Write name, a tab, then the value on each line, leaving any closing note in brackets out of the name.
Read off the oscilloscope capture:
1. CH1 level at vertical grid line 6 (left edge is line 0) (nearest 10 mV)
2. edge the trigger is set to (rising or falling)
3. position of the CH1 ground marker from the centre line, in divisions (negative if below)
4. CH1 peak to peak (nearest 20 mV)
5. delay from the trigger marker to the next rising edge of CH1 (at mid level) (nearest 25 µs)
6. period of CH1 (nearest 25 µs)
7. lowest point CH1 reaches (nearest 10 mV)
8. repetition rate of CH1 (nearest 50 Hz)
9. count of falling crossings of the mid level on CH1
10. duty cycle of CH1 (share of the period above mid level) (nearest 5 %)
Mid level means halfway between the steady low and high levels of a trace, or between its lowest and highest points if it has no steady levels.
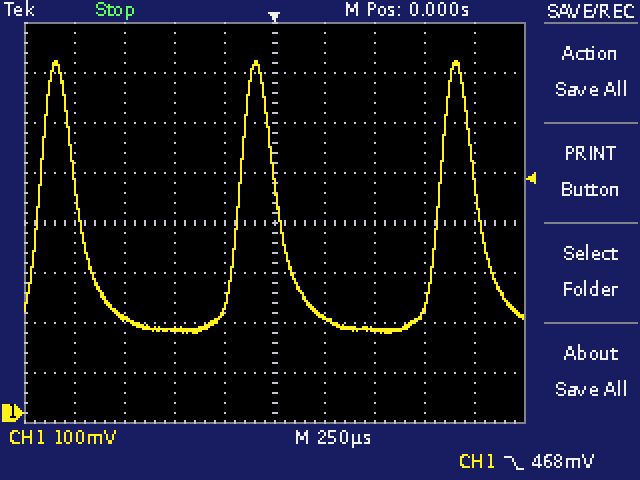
CH1 level at vertical grid line 6 (left edge is line 0)	190 mV
edge the trigger is set to	falling
position of the CH1 ground marker from the centre line, in divisions	-3.8 div
CH1 peak to peak	540 mV
delay from the trigger marker to the next rising edge of CH1 (at mid level)	825 µs
period of CH1	1.000 ms
lowest point CH1 reaches	160 mV
repetition rate of CH1	1.00 kHz
count of falling crossings of the mid level on CH1	3
duty cycle of CH1 (share of the period above mid level)	20 %
